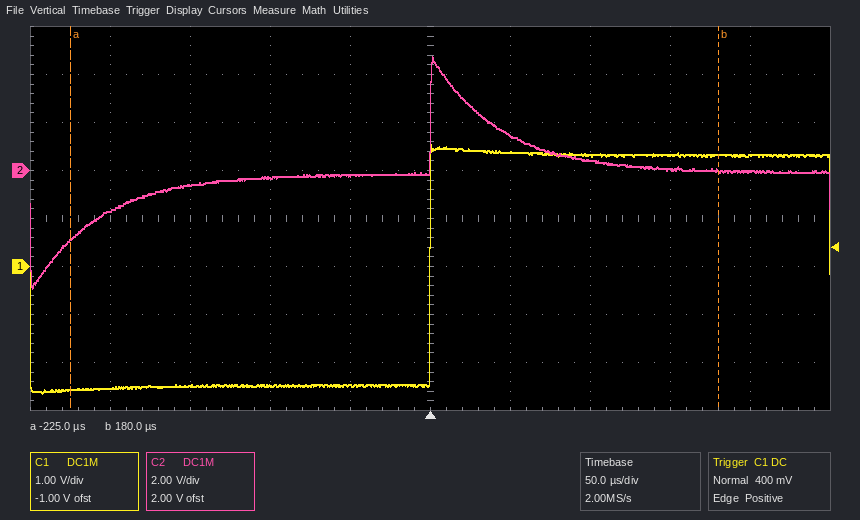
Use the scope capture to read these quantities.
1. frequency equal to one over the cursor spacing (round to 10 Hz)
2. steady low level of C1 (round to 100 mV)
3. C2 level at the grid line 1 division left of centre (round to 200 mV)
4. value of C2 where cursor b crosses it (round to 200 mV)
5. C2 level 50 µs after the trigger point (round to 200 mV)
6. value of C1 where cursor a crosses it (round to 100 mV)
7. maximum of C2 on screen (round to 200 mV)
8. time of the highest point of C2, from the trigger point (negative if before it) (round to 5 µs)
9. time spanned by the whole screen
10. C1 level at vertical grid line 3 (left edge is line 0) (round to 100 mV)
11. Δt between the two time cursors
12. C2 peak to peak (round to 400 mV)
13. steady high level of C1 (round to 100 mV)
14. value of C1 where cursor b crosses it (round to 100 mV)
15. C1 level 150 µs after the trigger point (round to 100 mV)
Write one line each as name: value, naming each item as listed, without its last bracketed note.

frequency equal to one over the cursor spacing: 2.47 kHz
steady low level of C1: -2.5 V
C2 level at the grid line 1 division left of centre: -200 mV
value of C2 where cursor b crosses it: 0.0 V
C2 level 50 µs after the trigger point: 1.4 V
value of C1 where cursor a crosses it: -2.6 V
maximum of C2 on screen: 4.8 V
time of the highest point of C2, from the trigger point (negative if before it): 0 µs
time spanned by the whole screen: 500 µs
C1 level at vertical grid line 3 (left edge is line 0): -2.5 V
Δt between the two time cursors: 405 µs
C2 peak to peak: 9.6 V
steady high level of C1: 2.3 V
value of C1 where cursor b crosses it: 2.3 V
C1 level 150 µs after the trigger point: 2.3 V
